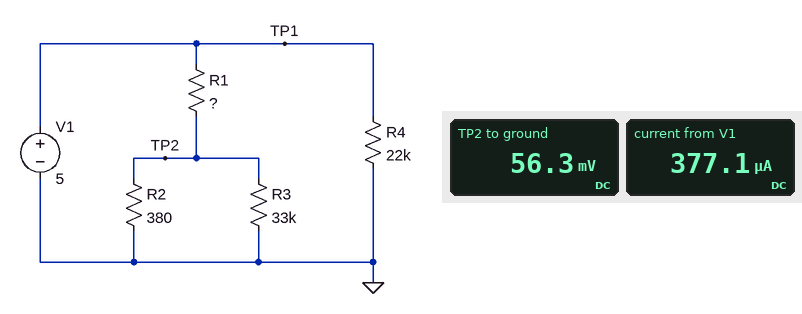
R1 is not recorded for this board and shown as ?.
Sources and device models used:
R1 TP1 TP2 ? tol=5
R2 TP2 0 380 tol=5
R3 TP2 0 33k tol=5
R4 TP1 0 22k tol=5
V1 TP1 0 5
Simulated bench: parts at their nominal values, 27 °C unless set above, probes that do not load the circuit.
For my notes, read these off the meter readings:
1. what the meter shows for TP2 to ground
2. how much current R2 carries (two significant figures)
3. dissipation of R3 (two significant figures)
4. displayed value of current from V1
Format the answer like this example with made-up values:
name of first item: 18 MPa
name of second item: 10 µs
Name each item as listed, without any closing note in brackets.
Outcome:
what the meter shows for TP2 to ground: 56.3 mV
how much current R2 carries: 150 µA
dissipation of R3: 96 nW
displayed value of current from V1: 377.1 µA
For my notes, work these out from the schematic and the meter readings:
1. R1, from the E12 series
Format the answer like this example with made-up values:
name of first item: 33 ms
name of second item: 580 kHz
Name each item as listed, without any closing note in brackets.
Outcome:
R1, from the E12 series: 33 kΩ
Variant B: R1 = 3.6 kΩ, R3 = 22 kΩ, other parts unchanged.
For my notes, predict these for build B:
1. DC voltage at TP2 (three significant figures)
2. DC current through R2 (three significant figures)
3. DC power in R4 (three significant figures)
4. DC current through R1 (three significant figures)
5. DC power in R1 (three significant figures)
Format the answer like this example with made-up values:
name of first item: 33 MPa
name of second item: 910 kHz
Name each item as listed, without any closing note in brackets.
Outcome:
DC voltage at TP2: 470 mV
DC current through R2: 1.24 mA
DC power in R4: 1.14 mW
DC current through R1: 1.26 mA
DC power in R1: 5.70 mW
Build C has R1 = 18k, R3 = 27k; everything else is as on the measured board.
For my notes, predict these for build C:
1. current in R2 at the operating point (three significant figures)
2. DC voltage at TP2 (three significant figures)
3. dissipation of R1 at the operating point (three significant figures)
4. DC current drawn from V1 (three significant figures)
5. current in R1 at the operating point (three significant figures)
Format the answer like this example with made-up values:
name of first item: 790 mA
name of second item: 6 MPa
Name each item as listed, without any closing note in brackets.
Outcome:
current in R2 at the operating point: 268 µA
DC voltage at TP2: 102 mV
dissipation of R1 at the operating point: 1.33 mW
DC current drawn from V1: 499 µA
current in R1 at the operating point: 272 µA
